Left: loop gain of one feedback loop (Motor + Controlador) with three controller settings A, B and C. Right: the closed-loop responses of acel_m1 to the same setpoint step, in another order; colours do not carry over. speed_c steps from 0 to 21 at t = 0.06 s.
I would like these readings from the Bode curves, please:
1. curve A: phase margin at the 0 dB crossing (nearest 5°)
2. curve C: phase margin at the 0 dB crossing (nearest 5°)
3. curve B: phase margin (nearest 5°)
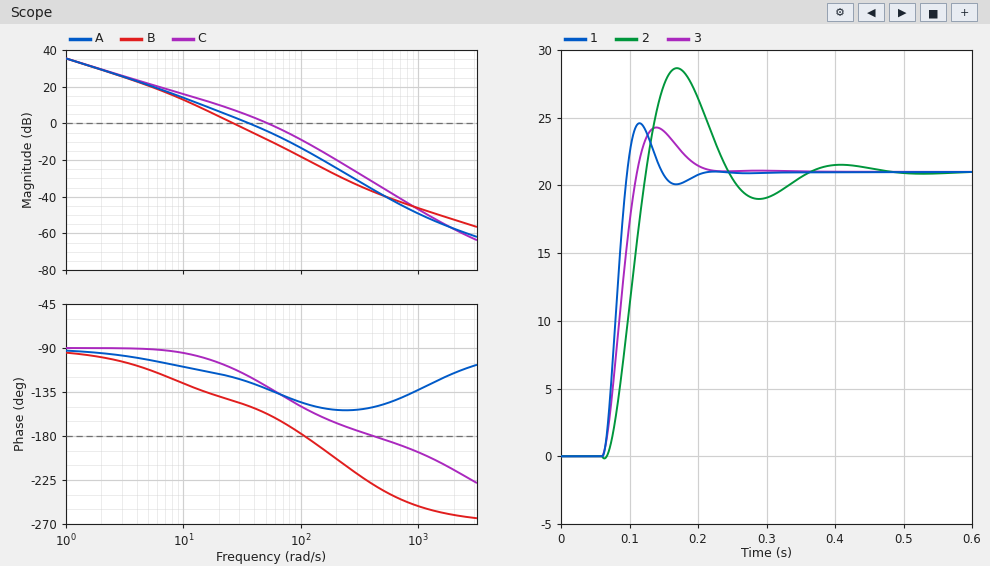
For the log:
55°
50°
35°
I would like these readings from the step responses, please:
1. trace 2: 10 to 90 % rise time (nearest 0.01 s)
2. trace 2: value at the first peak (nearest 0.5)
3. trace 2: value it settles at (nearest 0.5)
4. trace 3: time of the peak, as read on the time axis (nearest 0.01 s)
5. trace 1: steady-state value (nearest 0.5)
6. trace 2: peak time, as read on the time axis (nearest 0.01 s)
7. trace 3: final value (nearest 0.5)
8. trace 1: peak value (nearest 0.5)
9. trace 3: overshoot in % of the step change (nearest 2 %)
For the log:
0.04 s
28.5
21.0
0.14 s
21.0
0.17 s
21.0
24.5
16 %
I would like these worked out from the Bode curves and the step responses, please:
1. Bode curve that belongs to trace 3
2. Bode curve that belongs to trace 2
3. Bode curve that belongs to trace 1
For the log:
A
B
C
